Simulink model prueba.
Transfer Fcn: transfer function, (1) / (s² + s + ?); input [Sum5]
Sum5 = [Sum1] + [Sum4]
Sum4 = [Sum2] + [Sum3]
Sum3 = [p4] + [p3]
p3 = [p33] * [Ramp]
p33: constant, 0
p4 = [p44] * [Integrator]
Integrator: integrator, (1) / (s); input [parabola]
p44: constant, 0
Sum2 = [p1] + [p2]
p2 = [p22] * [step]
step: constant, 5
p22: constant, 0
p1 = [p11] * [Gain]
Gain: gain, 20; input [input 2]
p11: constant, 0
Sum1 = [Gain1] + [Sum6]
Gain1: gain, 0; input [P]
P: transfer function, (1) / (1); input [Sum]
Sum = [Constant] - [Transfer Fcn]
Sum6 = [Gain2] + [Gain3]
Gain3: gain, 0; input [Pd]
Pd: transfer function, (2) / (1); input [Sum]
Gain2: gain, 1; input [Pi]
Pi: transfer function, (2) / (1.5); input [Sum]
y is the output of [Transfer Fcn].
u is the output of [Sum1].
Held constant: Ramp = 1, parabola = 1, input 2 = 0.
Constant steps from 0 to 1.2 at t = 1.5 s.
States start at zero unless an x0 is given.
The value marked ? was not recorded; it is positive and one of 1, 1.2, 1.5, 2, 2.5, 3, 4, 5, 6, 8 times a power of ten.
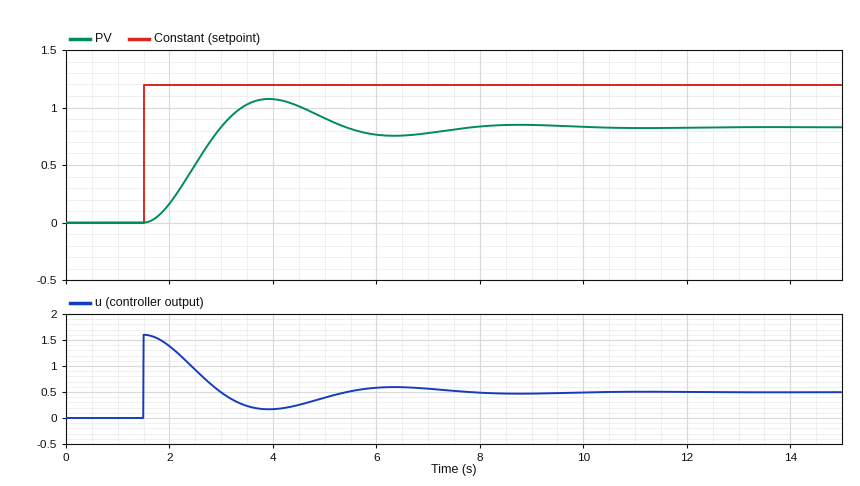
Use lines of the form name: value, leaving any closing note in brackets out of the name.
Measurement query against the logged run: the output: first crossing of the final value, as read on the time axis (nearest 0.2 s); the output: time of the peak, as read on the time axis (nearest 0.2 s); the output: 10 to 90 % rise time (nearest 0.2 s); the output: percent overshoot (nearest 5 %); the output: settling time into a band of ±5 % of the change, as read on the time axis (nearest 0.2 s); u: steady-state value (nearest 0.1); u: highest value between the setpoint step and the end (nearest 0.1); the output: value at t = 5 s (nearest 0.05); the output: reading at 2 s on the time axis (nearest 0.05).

the output: first crossing of the final value, as read on the time axis: 3.0 s
the output: time of the peak, as read on the time axis: 4.0 s
the output: 10 to 90 % rise time: 1.0 s
the output: percent overshoot: 30 %
the output: settling time into a band of ±5 % of the change, as read on the time axis: 7.2 s
u: steady-state value: 0.5
u: highest value between the setpoint step and the end: 1.6
the output: value at t = 5 s: 0.90
the output: reading at 2 s on the time axis: 0.15
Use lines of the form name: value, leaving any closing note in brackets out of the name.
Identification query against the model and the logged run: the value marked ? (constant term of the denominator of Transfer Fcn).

the value marked ?: 0.6
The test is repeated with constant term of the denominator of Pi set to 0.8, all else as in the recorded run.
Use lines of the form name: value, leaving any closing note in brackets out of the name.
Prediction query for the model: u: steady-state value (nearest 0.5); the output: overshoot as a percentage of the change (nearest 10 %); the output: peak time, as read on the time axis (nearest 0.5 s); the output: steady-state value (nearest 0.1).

u: steady-state value: 0.5
the output: overshoot as a percentage of the change: 40 %
the output: peak time, as read on the time axis: 3.5 s
the output: steady-state value: 1.0
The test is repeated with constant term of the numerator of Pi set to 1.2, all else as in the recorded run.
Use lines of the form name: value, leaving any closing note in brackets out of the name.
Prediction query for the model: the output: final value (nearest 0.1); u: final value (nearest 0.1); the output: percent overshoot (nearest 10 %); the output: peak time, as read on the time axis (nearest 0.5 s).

the output: final value: 0.7
u: final value: 0.4
the output: percent overshoot: 20 %
the output: peak time, as read on the time axis: 4.5 s
